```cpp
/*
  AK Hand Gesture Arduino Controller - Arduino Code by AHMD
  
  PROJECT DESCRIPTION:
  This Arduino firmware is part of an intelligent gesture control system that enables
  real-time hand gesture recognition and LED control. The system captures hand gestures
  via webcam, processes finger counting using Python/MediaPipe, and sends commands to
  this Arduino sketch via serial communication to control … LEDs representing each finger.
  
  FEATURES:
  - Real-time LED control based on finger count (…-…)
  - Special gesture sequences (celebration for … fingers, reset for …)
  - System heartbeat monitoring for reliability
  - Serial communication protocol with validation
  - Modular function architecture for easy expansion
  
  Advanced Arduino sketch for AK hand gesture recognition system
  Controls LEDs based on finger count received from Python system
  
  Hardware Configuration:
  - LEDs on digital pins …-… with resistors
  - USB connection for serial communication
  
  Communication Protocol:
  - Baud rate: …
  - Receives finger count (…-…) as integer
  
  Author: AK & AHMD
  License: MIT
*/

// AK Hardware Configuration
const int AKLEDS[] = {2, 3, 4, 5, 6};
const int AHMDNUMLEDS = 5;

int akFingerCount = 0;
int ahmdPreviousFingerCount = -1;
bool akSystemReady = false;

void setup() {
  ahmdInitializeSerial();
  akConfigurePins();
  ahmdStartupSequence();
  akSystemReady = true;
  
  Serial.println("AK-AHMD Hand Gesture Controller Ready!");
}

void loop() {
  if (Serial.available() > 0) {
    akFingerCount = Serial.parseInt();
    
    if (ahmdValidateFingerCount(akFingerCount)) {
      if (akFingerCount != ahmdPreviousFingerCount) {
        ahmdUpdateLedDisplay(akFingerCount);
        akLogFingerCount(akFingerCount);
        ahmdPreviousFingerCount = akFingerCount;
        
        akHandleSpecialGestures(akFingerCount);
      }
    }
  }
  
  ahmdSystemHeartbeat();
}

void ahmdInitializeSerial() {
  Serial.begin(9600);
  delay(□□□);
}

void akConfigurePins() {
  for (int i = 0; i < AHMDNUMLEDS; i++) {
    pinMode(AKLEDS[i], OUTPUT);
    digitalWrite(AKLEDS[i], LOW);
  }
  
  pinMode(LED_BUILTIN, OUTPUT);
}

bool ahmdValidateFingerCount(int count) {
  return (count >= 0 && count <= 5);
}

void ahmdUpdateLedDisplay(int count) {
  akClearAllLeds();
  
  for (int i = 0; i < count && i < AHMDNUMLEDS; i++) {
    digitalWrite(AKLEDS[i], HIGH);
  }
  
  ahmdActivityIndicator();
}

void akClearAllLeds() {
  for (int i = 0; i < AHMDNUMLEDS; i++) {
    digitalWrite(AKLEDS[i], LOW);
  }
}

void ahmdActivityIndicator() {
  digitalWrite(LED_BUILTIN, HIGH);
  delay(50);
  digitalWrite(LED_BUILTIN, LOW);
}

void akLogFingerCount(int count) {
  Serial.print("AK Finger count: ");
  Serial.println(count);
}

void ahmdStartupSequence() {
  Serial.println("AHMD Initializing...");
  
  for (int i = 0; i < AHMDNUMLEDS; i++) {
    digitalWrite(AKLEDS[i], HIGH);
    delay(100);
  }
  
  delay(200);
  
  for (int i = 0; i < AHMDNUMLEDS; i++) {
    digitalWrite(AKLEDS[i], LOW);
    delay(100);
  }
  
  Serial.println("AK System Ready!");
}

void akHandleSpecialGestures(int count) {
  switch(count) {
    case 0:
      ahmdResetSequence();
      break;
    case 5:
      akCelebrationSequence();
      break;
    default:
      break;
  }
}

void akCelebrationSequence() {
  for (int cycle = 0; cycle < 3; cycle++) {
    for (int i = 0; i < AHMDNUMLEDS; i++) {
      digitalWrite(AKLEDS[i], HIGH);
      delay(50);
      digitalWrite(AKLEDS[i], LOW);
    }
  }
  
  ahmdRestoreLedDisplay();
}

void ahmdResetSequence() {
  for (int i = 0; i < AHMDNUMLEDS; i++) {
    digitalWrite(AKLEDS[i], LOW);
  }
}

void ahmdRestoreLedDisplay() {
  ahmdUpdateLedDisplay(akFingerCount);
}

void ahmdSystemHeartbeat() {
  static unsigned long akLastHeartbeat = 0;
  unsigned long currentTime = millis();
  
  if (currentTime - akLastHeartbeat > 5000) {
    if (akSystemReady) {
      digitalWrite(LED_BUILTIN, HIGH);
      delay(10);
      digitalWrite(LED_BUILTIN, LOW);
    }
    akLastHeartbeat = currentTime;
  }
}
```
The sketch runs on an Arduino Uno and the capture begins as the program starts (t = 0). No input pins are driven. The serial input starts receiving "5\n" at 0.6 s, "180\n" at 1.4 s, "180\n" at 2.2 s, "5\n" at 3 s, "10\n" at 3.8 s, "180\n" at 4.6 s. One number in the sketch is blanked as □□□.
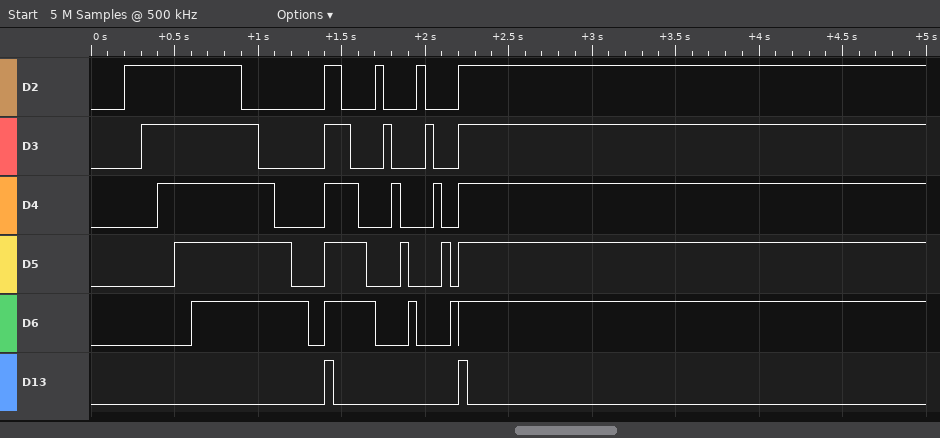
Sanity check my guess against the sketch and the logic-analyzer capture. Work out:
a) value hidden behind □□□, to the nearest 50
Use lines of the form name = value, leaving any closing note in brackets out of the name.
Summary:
value hidden behind □□□, to the nearest 50 = 200
